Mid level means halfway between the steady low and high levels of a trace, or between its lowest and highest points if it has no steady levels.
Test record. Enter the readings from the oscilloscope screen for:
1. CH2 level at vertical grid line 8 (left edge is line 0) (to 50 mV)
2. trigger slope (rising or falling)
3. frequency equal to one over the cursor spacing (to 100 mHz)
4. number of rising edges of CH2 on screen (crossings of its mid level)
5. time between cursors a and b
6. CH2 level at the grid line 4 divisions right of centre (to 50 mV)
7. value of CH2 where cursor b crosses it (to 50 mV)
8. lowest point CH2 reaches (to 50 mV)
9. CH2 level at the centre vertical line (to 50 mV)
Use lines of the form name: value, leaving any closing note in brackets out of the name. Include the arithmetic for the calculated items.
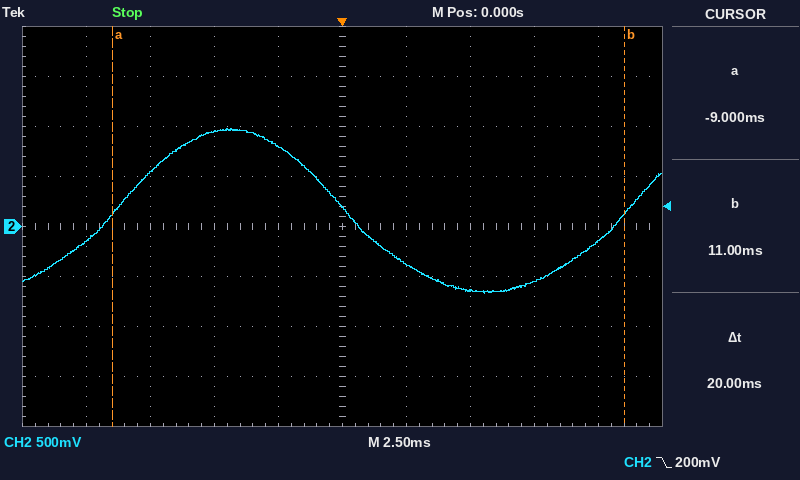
CH2 level at vertical grid line 8 (left edge is line 0): -550 mV
trigger slope: falling
frequency equal to one over the cursor spacing: 1 / 20 ms ≈ 50.0 Hz
number of rising edges of CH2 on screen: 2
time between cursors a and b: 20 ms
CH2 level at the grid line 4 divisions right of centre: -150 mV
value of CH2 where cursor b crosses it: 150 mV
lowest point CH2 reaches: -650 mV
CH2 level at the centre vertical line: 200 mV
